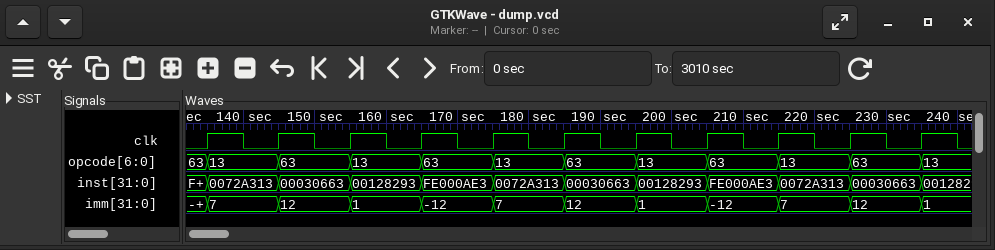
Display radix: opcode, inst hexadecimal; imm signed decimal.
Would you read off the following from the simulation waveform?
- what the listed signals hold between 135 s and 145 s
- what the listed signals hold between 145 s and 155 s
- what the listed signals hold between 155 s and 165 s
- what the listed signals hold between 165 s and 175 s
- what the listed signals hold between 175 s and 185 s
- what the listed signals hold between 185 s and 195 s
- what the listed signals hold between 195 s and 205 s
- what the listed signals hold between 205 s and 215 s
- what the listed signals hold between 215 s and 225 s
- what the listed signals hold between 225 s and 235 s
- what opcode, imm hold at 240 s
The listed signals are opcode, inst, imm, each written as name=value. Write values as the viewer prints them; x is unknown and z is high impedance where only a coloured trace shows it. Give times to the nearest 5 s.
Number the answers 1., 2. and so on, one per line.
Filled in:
1. opcode=13, inst=0072A313, imm=7
2. opcode=63, inst=00030663, imm=12
3. opcode=13, inst=00128293, imm=1
4. opcode=63, inst=FE000AE3, imm=-12
5. opcode=13, inst=0072A313, imm=7
6. opcode=63, inst=00030663, imm=12
7. opcode=13, inst=00128293, imm=1
8. opcode=63, inst=FE000AE3, imm=-12
9. opcode=13, inst=0072A313, imm=7
10. opcode=63, inst=00030663, imm=12
11. opcode=13, imm=1
